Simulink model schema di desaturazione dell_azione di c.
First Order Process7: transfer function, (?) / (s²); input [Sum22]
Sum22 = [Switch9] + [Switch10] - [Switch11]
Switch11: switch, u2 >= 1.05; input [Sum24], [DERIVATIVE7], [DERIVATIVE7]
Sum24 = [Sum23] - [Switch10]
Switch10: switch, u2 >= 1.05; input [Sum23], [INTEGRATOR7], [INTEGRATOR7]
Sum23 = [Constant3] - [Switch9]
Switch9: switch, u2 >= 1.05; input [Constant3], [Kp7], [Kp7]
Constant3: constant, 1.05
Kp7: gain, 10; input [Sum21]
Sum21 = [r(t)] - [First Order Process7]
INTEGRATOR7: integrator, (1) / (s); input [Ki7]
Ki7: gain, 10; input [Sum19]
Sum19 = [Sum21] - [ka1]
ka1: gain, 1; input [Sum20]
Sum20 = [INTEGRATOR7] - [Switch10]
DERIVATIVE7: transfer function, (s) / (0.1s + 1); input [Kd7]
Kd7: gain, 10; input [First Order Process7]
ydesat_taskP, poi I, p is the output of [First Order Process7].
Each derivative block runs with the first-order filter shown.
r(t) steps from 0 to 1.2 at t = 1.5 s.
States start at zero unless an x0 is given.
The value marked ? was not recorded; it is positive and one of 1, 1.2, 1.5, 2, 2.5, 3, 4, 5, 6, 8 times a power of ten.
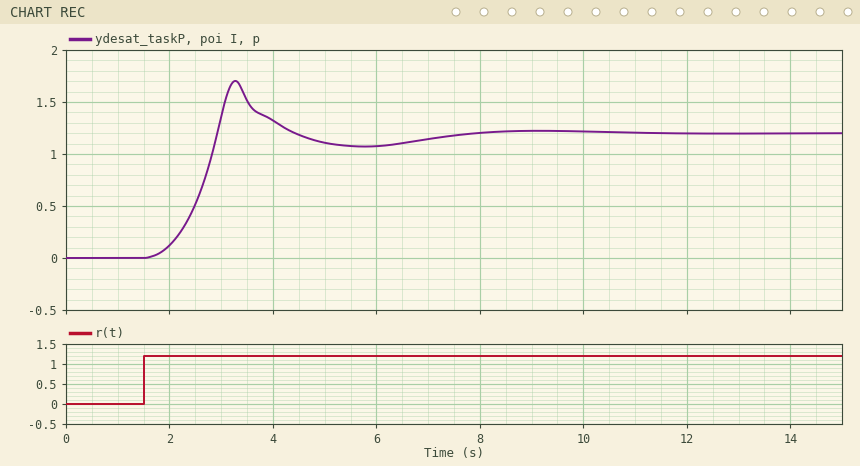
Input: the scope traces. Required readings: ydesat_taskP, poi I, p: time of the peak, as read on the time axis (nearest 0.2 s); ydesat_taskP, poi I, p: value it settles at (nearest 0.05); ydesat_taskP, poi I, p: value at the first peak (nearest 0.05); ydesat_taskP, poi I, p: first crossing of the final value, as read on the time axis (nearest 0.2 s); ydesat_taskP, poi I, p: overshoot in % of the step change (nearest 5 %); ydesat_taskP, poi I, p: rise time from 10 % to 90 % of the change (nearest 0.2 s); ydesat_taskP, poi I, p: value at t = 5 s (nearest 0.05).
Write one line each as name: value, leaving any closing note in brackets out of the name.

ydesat_taskP, poi I, p: time of the peak, as read on the time axis: 3.2 s
ydesat_taskP, poi I, p: value it settles at: 1.20
ydesat_taskP, poi I, p: value at the first peak: 1.70
ydesat_taskP, poi I, p: first crossing of the final value, as read on the time axis: 3.0 s
ydesat_taskP, poi I, p: overshoot in % of the step change: 40 %
ydesat_taskP, poi I, p: rise time from 10 % to 90 % of the change: 0.8 s
ydesat_taskP, poi I, p: value at t = 5 s: 1.10
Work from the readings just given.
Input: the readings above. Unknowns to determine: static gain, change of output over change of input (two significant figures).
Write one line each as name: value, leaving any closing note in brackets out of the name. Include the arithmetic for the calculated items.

static gain, change of output over change of input: (1.2 - 0) / (1.2 - 0) = 1.0
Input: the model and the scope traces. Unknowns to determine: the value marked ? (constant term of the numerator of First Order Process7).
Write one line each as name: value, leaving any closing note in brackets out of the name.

the value marked ?: 1
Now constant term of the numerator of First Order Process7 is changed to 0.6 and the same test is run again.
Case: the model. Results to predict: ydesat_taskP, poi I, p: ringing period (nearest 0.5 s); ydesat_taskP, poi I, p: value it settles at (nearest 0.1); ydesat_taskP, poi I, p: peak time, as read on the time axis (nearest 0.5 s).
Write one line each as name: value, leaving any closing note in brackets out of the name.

ydesat_taskP, poi I, p: ringing period: 4.0 s
ydesat_taskP, poi I, p: value it settles at: 1.2
ydesat_taskP, poi I, p: peak time, as read on the time axis: 4.0 s
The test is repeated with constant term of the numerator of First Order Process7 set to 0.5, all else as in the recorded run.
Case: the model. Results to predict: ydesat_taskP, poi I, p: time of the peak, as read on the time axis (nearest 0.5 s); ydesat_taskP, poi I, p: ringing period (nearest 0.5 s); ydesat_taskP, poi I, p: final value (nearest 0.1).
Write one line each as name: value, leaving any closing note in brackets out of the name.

ydesat_taskP, poi I, p: time of the peak, as read on the time axis: 4.0 s
ydesat_taskP, poi I, p: ringing period: 4.0 s
ydesat_taskP, poi I, p: final value: 1.2
